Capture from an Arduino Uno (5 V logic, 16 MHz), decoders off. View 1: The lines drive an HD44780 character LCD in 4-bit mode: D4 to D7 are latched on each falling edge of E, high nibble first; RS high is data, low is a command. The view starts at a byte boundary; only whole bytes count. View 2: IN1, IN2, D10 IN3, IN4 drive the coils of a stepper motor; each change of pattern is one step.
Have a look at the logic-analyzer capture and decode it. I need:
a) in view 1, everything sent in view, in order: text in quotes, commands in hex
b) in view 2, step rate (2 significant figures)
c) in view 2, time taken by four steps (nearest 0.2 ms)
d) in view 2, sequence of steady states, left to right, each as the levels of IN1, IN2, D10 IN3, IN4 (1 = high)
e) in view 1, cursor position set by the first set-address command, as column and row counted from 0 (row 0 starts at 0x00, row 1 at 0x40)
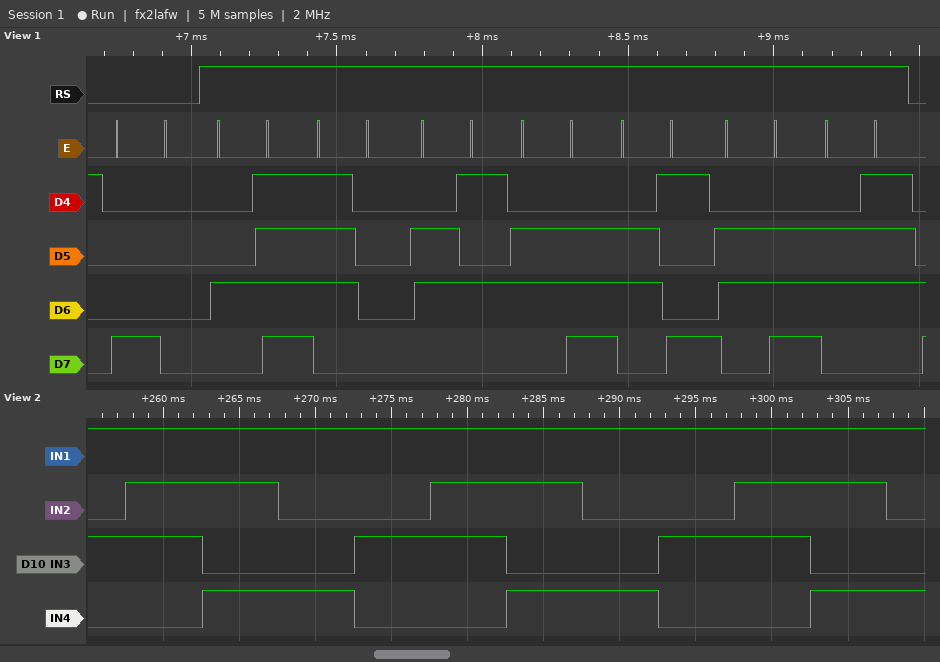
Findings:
0x80 "Opening"
200 steps/s
20.0 ms
1010 1110 1101 1001 1010 1110 1101 1001 1010 1110 1101 1001
column 0, row 0
